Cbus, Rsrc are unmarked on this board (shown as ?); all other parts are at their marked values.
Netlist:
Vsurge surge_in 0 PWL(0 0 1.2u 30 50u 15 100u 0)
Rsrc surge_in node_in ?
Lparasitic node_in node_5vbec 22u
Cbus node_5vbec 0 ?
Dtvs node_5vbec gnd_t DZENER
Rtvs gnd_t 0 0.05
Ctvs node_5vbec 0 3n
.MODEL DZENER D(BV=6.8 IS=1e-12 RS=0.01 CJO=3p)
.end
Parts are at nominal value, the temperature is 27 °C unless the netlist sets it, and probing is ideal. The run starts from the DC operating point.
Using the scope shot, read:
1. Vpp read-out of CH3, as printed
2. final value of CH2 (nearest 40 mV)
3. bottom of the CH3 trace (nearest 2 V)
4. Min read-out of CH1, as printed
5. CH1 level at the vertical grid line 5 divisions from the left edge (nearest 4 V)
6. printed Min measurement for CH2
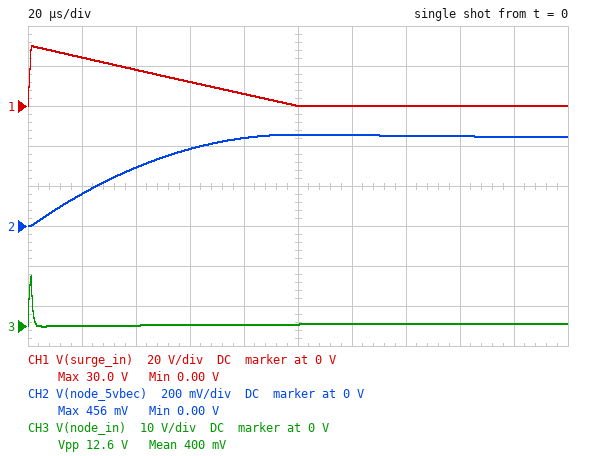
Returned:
12.6 V
440 mV
0 V
0.00 V
0 V
0.00 V
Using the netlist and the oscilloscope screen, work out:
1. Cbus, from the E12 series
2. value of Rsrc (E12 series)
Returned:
82 µF
39 Ω
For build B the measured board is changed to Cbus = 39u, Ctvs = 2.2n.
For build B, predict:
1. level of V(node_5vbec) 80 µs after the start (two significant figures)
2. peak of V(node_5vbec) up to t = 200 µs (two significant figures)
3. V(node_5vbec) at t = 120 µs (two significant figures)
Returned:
680 mV
700 mV
620 mV
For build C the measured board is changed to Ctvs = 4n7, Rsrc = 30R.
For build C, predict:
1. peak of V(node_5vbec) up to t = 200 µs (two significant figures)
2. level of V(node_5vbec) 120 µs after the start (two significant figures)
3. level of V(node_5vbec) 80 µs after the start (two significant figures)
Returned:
590 mV
580 mV
570 mV
